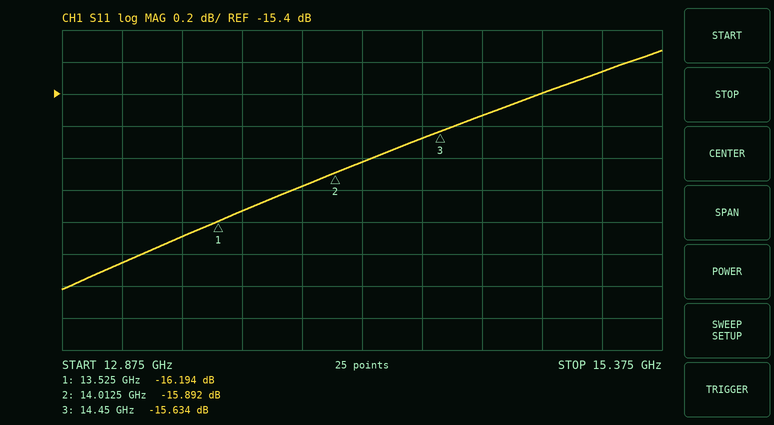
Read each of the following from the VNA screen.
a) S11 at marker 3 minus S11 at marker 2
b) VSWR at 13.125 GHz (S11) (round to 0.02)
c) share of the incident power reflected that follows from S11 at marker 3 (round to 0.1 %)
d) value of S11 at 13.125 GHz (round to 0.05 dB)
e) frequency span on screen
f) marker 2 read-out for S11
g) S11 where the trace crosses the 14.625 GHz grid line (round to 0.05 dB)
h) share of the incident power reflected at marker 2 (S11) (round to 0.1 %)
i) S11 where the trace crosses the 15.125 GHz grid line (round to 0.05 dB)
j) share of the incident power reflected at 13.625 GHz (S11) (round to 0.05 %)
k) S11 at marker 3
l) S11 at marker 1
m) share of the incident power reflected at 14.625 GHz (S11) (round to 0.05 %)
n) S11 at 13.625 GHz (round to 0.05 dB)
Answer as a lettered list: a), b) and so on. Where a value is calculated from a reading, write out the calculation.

a) -15.634 − (-15.892) = 0.258 dB
b) |Γ| = 10^(-16.45/20) = 0.1505; VSWR = (1 + 0.1505)/(1 − 0.1505) ≈ 1.35, so 1.36 to the nearest 0.02
c) 10^(-15.634/10) ≈ 2.7 %
d) -16.45 dB
e) 2.5 GHz
f) -15.892 dB
g) -15.55 dB
h) 10^(-15.892/10) ≈ 2.6 %
i) -15.25 dB
j) 10^(-16.15/10) ≈ 2.43 %, so 2.45 % to the nearest 0.05 %
k) -15.634 dB
l) -16.194 dB
m) 10^(-15.55/10) ≈ 2.79 %, so 2.80 % to the nearest 0.05 %
n) -16.15 dB
